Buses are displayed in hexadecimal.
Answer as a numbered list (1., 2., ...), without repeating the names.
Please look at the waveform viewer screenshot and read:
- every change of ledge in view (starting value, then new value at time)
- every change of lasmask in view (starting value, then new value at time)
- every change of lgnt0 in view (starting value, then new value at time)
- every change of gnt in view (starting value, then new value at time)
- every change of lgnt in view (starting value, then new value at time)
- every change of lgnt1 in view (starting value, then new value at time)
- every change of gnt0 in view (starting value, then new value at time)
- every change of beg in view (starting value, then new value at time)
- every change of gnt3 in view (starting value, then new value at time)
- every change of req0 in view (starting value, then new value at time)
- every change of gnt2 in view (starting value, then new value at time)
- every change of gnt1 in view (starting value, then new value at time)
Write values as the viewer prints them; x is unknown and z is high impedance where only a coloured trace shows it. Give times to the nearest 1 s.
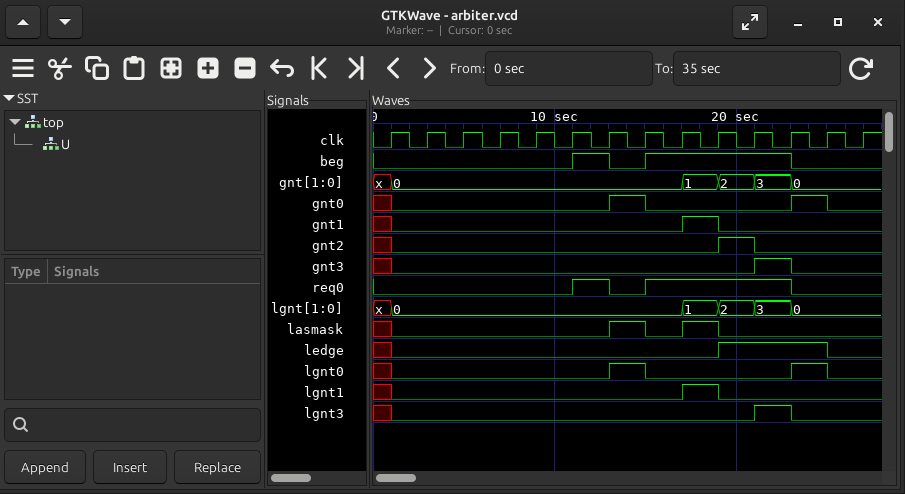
1. x, 0 at 1 s, 1 at 19 s, 0 at 25 s
2. x, 0 at 1 s, 1 at 13 s, 0 at 15 s, 1 at 17 s, 0 at 19 s
3. x, 0 at 1 s, 1 at 13 s, 0 at 15 s, 1 at 23 s, 0 at 25 s
4. x, 0 at 1 s, 1 at 17 s, 2 at 19 s, 3 at 21 s, 0 at 23 s
5. x, 0 at 1 s, 1 at 17 s, 2 at 19 s, 3 at 21 s, 0 at 23 s
6. x, 0 at 1 s, 1 at 17 s, 0 at 19 s
7. x, 0 at 1 s, 1 at 13 s, 0 at 15 s, 1 at 23 s, 0 at 25 s
8. 0, 1 at 11 s, 0 at 13 s, 1 at 15 s, 0 at 23 s
9. x, 0 at 1 s, 1 at 21 s, 0 at 23 s
10. 0, 1 at 11 s, 0 at 13 s, 1 at 15 s, 0 at 23 s
11. x, 0 at 1 s, 1 at 19 s, 0 at 21 s
12. x, 0 at 1 s, 1 at 17 s, 0 at 19 s
